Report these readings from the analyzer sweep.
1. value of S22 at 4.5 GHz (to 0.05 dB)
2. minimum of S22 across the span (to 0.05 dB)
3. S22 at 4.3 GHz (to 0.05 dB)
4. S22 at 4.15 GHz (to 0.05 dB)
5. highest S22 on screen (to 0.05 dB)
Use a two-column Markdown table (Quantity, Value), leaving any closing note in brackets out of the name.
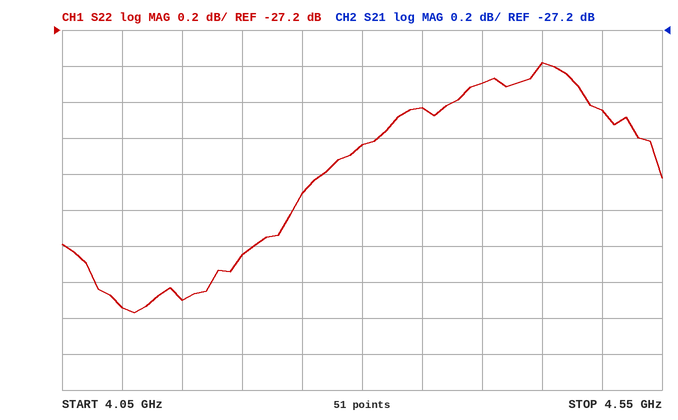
| Quantity | Value |
|---|---|
| value of S22 at 4.5 GHz | -27.65 dB |
| minimum of S22 across the span | -28.75 dB |
| S22 at 4.3 GHz | -27.85 dB |
| S22 at 4.15 GHz | -28.70 dB |
| highest S22 on screen | -27.40 dB |
